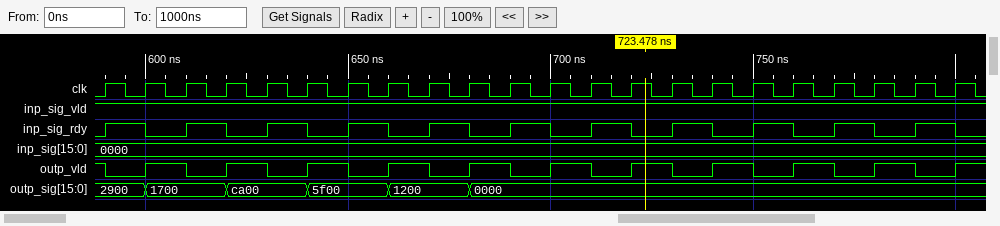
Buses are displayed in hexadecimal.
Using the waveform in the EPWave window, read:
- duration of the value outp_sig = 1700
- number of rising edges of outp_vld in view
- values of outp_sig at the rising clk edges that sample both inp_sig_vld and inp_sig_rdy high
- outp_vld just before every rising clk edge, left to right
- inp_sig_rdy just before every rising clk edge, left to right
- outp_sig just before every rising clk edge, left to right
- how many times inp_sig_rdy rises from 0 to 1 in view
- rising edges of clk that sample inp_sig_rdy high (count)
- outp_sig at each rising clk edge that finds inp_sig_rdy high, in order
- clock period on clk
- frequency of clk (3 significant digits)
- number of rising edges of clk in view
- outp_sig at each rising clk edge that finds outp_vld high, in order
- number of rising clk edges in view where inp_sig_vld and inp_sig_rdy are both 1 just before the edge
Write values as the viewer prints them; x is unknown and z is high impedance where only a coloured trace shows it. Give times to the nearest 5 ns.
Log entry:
20 ns
11
2900, 1700, ca00, 5f00, 1200, 0000, 0000, 0000, 0000, 0000, 0000
1 0 1 0 1 0 1 0 1 0 1 0 1 0 1 0 1 0 1 0 1 0
0 1 0 1 0 1 0 1 0 1 0 1 0 1 0 1 0 1 0 1 0 1
2900, 2900, 1700, 1700, ca00, ca00, 5f00, 5f00, 1200, 1200, 0000, 0000, 0000, 0000, 0000, 0000, 0000, 0000, 0000, 0000, 0000, 0000
11
11
2900, 1700, ca00, 5f00, 1200, 0000, 0000, 0000, 0000, 0000, 0000
10 ns
100 MHz
22
2900, 1700, ca00, 5f00, 1200, 0000, 0000, 0000, 0000, 0000, 0000
11
